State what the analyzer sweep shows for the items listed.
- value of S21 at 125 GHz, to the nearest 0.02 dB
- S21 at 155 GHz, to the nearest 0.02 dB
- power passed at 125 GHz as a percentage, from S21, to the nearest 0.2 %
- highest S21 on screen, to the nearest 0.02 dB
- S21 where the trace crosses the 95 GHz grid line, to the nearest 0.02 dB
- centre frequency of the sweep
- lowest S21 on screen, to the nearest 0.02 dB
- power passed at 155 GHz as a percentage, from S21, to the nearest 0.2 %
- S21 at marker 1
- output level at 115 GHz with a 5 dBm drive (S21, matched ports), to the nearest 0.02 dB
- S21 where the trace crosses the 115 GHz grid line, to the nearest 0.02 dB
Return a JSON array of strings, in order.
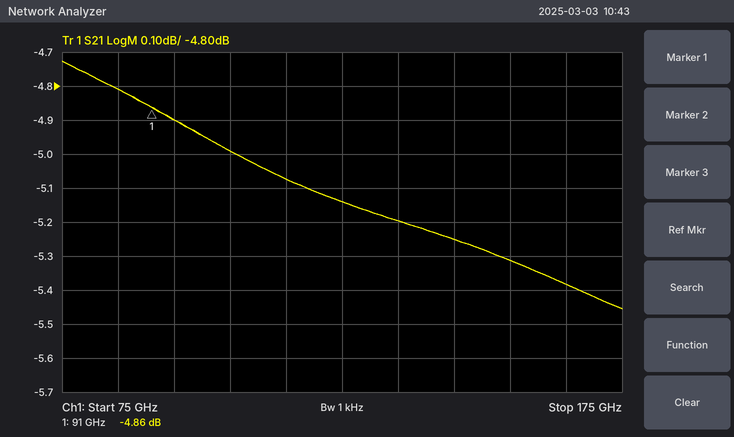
["-5.14 dB", "-5.32 dB", "30.6 %", "-4.72 dB", "-4.90 dB", "125 GHz", "-5.46 dB", "29.4 %", "-4.86 dB", "-0.08 dBm", "-5.08 dB"]
